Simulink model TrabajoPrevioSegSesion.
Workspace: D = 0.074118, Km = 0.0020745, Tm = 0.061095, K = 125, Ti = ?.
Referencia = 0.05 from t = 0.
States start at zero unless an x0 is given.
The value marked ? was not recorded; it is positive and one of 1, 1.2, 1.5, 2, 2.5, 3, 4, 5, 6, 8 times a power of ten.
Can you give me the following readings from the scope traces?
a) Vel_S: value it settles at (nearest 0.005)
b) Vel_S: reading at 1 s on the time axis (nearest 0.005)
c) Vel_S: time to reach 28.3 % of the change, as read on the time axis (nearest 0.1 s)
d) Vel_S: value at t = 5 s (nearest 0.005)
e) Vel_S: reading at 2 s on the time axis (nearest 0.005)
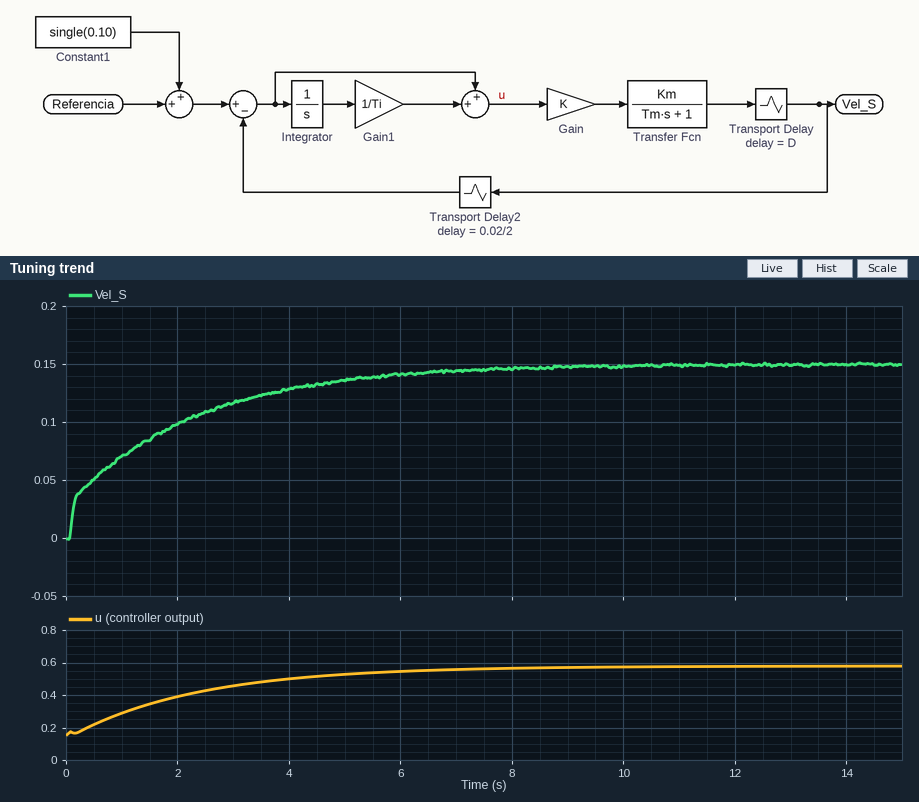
0.150
0.070
0.3 s
0.135
0.100
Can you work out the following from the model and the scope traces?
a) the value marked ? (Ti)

0.5
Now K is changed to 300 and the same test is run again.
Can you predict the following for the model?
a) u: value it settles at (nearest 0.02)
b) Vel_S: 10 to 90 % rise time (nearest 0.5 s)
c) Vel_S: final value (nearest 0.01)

0.24
2.0 s
0.15
